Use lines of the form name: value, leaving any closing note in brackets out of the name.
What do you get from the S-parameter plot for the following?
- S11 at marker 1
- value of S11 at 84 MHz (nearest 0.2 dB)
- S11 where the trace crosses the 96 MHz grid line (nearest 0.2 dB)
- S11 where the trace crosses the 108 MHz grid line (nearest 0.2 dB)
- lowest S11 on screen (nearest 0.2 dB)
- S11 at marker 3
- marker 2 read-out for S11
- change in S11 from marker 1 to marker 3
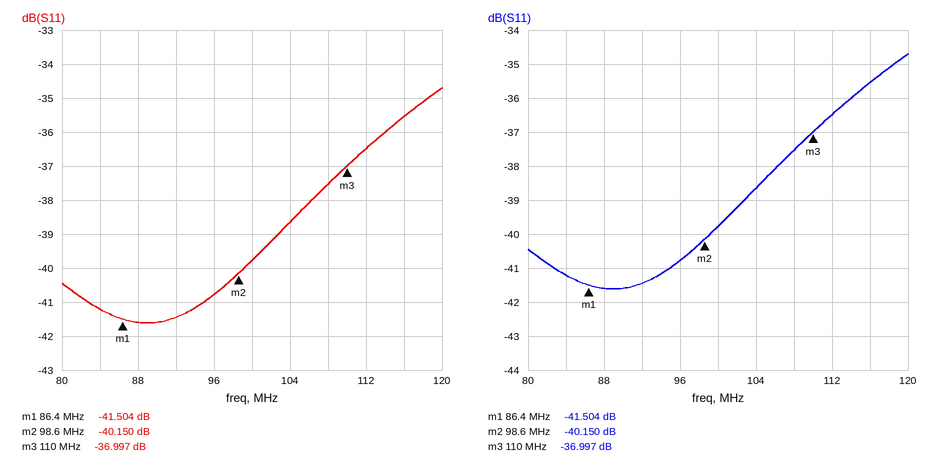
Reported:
S11 at marker 1: -41.504 dB
value of S11 at 84 MHz: -41.2 dB
S11 where the trace crosses the 96 MHz grid line: -40.8 dB
S11 where the trace crosses the 108 MHz grid line: -37.6 dB
lowest S11 on screen: -41.6 dB
S11 at marker 3: -36.997 dB
marker 2 read-out for S11: -40.150 dB
change in S11 from marker 1 to marker 3: 4.507 dB
